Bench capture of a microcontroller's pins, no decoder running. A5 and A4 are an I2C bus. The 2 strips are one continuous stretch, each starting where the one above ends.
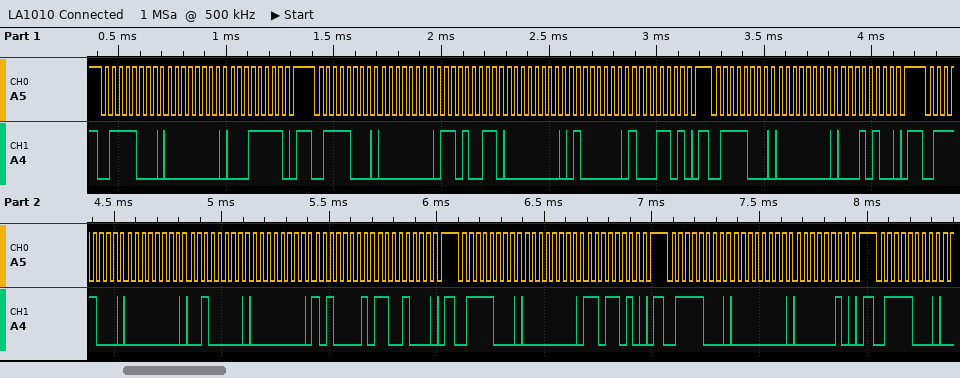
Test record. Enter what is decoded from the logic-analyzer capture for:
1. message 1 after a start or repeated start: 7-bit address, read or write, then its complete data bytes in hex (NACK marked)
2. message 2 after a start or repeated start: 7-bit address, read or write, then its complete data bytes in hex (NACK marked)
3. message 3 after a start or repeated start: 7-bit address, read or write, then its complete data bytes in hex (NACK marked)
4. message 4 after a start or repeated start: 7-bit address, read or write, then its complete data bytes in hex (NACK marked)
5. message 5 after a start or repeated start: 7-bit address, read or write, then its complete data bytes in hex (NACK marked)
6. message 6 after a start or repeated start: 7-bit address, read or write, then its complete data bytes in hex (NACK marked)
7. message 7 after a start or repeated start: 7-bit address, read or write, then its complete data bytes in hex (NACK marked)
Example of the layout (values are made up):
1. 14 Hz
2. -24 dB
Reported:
1. 0x3C write: 00 1F
2. 0x3C write: 00 D3 00 40 8D
3. 0x3C write: 00 14
4. 0x3C write: 00 20 00 A1 C8
5. 0x3C write: 00 DA
6. 0x3C write: 00 02
7. 0x3C write
